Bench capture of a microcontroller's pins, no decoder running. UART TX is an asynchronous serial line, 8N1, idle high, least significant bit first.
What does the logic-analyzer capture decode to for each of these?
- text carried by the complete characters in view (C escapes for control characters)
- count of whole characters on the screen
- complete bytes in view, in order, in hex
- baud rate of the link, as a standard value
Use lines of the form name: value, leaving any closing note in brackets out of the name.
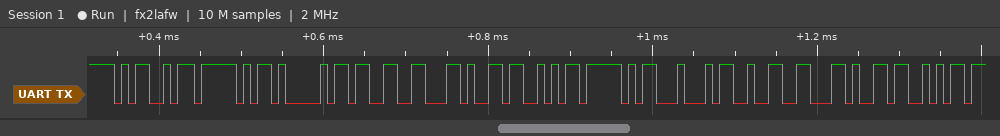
text carried by the complete characters in view: "M_A3,S_D2,S"
count of whole characters on the screen: 11
complete bytes in view, in order, in hex: 0x4D 0x5F 0x41 0x33 0x2C 0x53 0x5F 0x44 0x32 0x2C 0x53
baud rate of the link, as a standard value: 115200 baud
